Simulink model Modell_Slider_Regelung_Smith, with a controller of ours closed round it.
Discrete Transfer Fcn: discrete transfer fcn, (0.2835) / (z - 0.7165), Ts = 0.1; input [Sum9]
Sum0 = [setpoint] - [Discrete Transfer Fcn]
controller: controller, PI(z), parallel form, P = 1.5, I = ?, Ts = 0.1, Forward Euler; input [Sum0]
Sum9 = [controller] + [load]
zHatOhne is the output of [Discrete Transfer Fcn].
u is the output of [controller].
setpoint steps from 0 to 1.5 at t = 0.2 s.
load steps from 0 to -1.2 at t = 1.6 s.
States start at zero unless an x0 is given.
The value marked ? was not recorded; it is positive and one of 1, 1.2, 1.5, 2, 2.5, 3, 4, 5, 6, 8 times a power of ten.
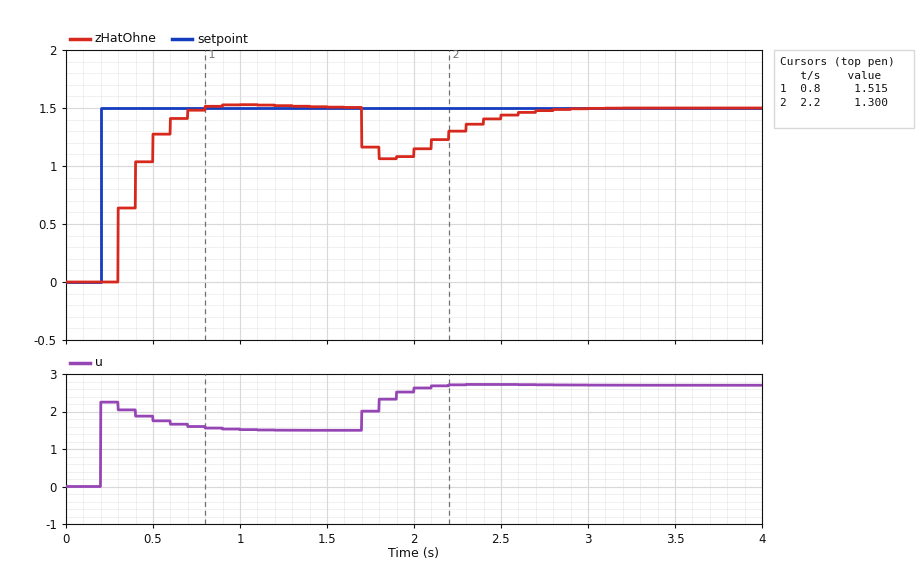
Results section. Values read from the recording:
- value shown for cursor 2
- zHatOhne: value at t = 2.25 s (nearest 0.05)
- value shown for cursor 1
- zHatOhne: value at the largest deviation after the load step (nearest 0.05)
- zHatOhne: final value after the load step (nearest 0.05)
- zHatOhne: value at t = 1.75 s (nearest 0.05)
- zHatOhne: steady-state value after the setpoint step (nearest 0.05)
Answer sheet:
1.300
1.30
1.515
1.05
1.50
1.15
1.50
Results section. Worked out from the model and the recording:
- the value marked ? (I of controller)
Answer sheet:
5
